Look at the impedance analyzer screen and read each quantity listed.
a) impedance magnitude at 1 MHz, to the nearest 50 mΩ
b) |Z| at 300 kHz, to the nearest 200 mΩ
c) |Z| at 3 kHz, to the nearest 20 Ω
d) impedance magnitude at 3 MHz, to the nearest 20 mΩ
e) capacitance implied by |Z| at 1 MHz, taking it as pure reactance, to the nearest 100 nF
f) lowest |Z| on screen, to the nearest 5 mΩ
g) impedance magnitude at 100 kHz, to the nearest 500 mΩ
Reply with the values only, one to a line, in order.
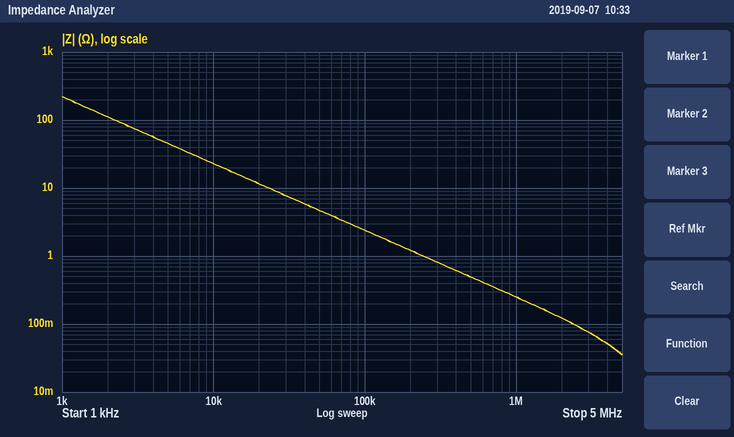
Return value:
250 mΩ
800 mΩ
80 Ω
80 mΩ
600 nF
35 mΩ
2.5 Ω
